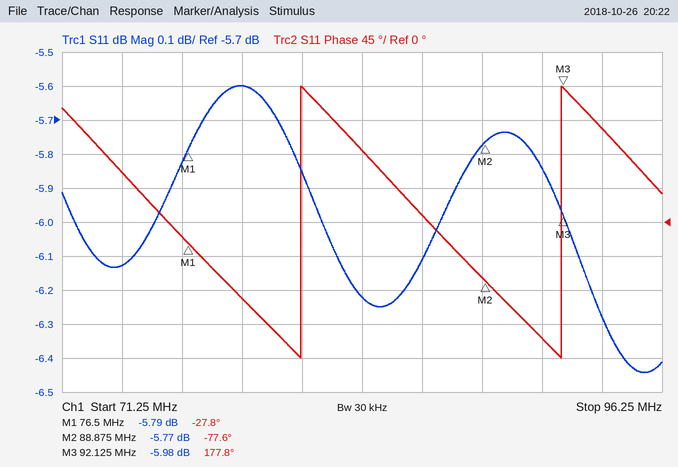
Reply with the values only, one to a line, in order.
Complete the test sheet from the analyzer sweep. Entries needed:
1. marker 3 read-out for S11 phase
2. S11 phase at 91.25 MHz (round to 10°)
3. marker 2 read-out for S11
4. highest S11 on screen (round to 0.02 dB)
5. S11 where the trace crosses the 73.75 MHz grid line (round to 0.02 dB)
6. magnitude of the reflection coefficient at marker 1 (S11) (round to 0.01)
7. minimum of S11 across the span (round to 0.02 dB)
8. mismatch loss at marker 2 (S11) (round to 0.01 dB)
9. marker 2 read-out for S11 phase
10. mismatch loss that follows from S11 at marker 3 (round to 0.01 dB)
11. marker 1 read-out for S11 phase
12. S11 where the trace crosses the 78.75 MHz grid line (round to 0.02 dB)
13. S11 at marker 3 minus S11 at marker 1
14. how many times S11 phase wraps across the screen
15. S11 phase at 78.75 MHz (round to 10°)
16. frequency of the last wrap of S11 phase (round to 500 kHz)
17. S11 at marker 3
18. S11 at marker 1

177.8°
-150°
-5.77 dB
-5.60 dB
-6.12 dB
0.51
-6.44 dB
1.34 dB
-77.6°
1.26 dB
-27.8°
-5.60 dB
-0.19 dB
2
-100°
92.0 MHz
-5.98 dB
-5.79 dB
